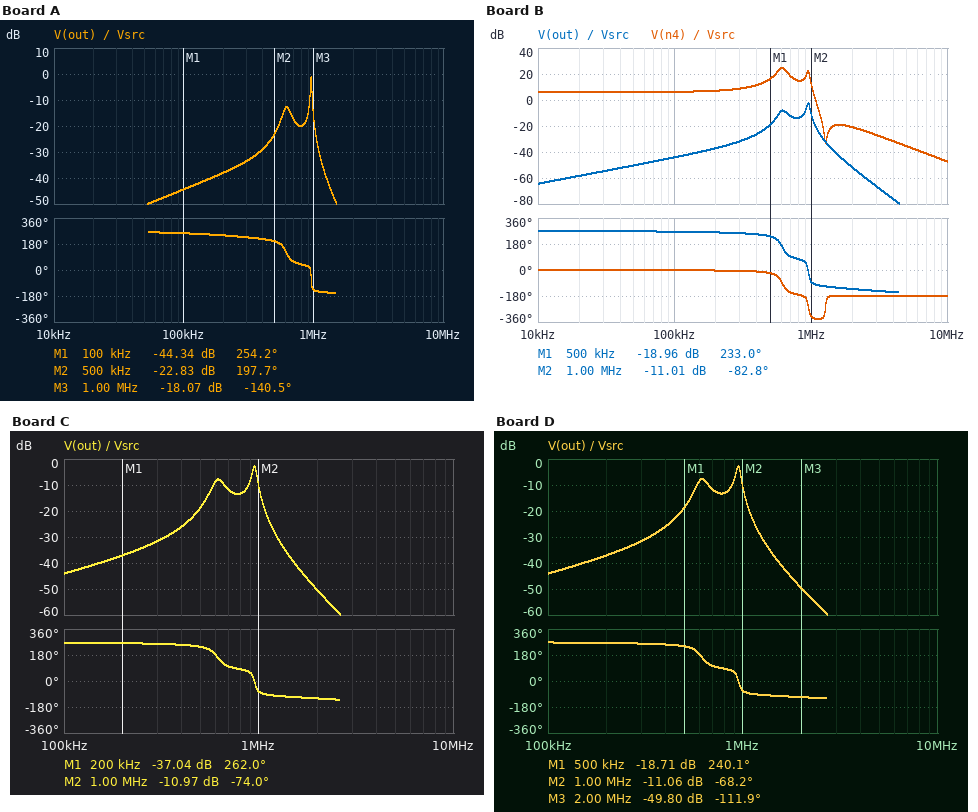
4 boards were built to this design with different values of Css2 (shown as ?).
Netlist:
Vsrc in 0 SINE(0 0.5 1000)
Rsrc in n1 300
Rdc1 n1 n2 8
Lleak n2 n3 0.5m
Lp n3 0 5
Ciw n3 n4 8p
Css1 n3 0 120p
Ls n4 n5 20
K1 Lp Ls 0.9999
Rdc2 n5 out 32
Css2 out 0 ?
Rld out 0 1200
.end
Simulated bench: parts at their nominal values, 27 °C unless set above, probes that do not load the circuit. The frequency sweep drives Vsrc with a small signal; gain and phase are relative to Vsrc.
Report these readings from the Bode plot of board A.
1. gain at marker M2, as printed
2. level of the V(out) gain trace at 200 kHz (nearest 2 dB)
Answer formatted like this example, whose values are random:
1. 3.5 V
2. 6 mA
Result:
1. -22.83 dB
2. -38 dB
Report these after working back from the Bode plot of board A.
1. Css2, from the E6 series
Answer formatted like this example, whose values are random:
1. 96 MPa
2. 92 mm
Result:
1. 330 pF
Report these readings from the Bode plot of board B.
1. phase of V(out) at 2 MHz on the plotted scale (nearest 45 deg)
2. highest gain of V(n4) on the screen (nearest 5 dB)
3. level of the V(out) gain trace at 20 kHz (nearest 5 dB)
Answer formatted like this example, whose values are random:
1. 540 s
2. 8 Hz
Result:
1. -135 deg
2. 25 dB
3. -60 dB
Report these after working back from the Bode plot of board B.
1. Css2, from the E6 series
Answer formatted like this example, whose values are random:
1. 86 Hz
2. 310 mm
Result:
1. 68 pF
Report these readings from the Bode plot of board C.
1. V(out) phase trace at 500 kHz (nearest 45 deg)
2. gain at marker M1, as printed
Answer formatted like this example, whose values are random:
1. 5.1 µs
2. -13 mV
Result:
1. 225 deg
2. -37.04 dB
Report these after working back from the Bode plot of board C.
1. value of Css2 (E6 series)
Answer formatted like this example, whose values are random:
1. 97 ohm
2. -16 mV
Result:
1. 47 pF
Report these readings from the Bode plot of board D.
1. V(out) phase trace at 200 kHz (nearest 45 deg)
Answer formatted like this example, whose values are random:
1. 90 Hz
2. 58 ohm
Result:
1. 270 deg
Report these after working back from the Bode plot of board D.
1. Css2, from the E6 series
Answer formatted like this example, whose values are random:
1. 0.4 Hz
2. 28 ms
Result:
1. 33 pF
